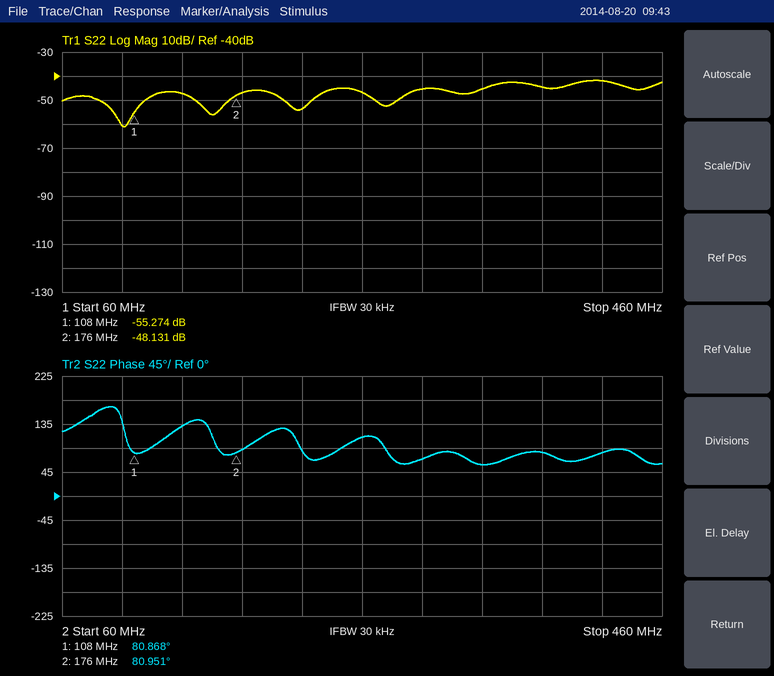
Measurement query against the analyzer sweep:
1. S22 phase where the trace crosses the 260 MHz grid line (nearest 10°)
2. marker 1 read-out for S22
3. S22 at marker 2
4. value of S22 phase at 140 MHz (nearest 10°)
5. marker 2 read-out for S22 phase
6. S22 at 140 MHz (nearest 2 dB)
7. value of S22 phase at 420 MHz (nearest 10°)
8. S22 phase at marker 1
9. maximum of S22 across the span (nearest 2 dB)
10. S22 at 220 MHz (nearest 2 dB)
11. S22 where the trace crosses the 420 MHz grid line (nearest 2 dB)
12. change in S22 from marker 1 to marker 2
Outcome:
110°
-55.274 dB
-48.131 dB
130°
80.951°
-48 dB
80°
80.868°
-42 dB
-54 dB
-42 dB
7.143 dB
